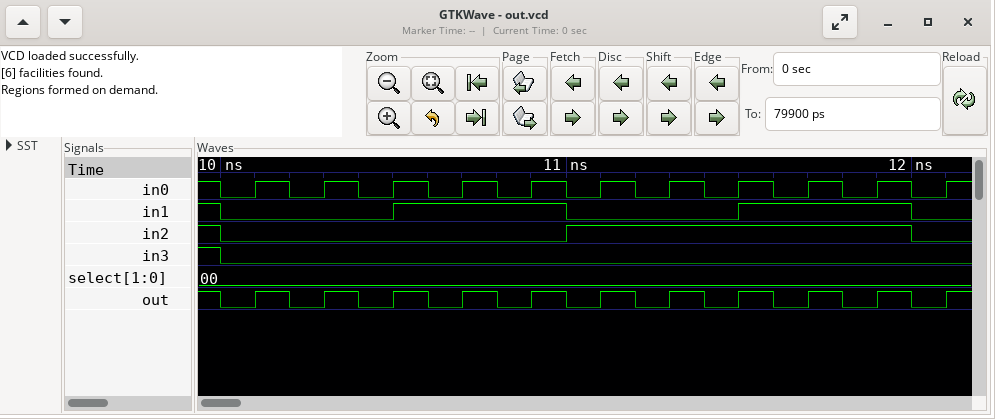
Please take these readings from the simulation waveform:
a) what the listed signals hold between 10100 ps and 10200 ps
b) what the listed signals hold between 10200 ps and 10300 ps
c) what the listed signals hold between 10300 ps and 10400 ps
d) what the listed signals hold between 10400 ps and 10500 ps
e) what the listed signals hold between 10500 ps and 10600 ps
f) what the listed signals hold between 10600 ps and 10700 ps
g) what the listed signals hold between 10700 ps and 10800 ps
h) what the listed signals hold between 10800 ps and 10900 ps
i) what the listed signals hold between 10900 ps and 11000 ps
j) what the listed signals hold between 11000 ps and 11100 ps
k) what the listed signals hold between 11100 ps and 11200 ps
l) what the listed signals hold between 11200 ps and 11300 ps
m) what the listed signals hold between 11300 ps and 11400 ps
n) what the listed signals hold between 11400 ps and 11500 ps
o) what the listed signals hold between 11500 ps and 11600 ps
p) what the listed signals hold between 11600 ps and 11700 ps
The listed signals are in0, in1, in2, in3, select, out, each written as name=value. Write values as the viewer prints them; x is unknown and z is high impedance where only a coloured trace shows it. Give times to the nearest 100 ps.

in0=1, in1=0, in2=0, in3=0, select=00, out=1
in0=0, in1=0, in2=0, in3=0, select=00, out=0
in0=1, in1=0, in2=0, in3=0, select=00, out=1
in0=0, in1=0, in2=0, in3=0, select=00, out=0
in0=1, in1=1, in2=0, in3=0, select=00, out=1
in0=0, in1=1, in2=0, in3=0, select=00, out=0
in0=1, in1=1, in2=0, in3=0, select=00, out=1
in0=0, in1=1, in2=0, in3=0, select=00, out=0
in0=1, in1=1, in2=0, in3=0, select=00, out=1
in0=0, in1=0, in2=1, in3=0, select=00, out=0
in0=1, in1=0, in2=1, in3=0, select=00, out=1
in0=0, in1=0, in2=1, in3=0, select=00, out=0
in0=1, in1=0, in2=1, in3=0, select=00, out=1
in0=0, in1=0, in2=1, in3=0, select=00, out=0
in0=1, in1=1, in2=1, in3=0, select=00, out=1
in0=0, in1=1, in2=1, in3=0, select=00, out=0
